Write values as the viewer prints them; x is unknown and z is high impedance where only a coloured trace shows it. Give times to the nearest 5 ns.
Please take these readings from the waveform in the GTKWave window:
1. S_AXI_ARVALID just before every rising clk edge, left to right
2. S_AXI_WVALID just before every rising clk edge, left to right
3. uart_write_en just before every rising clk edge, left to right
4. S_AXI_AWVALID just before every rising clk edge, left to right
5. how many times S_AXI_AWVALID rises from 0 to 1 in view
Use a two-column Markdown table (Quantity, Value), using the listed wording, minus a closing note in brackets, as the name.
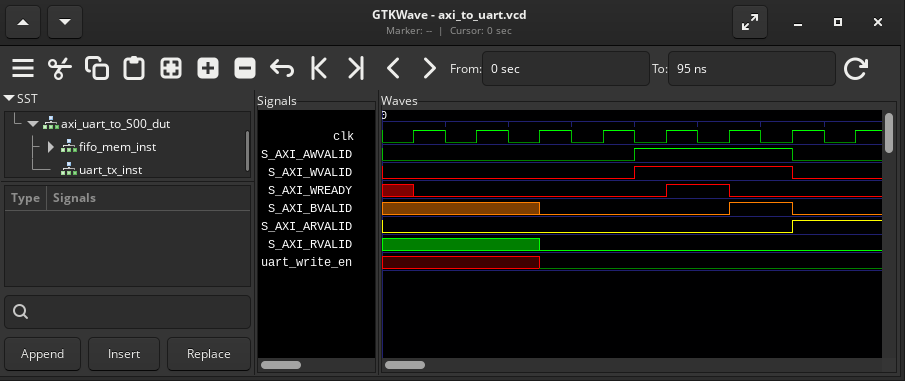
| Quantity | Value |
|---|---|
| S_AXI_ARVALID just before every rising clk edge, left to right | 0 0 0 0 0 0 0 1 |
| S_AXI_WVALID just before every rising clk edge, left to right | 0 0 0 0 1 1 1 0 |
| uart_write_en just before every rising clk edge, left to right | x x x 0 0 0 0 0 |
| S_AXI_AWVALID just before every rising clk edge, left to right | 0 0 0 0 1 1 1 0 |
| how many times S_AXI_AWVALID rises from 0 to 1 in view | 1 |
